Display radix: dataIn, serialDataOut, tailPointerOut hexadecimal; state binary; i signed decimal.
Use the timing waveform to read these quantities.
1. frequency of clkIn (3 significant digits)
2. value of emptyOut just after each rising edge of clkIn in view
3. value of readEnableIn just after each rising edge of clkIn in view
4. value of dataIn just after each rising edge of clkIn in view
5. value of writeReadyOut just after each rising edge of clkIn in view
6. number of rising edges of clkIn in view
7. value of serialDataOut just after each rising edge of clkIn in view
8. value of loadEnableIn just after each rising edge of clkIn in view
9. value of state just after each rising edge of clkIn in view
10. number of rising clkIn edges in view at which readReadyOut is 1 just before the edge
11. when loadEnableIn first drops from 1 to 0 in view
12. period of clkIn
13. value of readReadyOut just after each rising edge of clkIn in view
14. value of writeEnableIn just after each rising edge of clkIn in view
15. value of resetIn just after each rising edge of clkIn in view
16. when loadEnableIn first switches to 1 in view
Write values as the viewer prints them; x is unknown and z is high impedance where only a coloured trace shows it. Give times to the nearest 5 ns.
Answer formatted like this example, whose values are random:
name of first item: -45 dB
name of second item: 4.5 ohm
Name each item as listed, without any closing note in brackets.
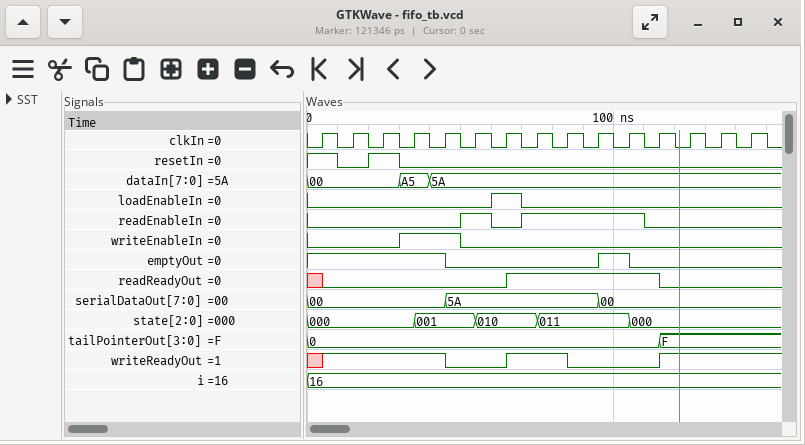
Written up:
frequency of clkIn: 100 MHz
value of emptyOut just after each rising edge of clkIn in view: 1 1 1 1 0 0 0 0 0 1 0 0 0 0 0
value of readEnableIn just after each rising edge of clkIn in view: 0 0 0 0 0 1 0 1 1 1 1 0 0 0 0
value of dataIn just after each rising edge of clkIn in view: 00, 00, 00, A5, 5A, 5A, 5A, 5A, 5A, 5A, 5A, 5A, 5A, 5A, 5A
value of writeReadyOut just after each rising edge of clkIn in view: 1 1 1 1 0 0 1 1 0 0 0 1 1 1 1
number of rising edges of clkIn in view: 15
value of serialDataOut just after each rising edge of clkIn in view: 00, 00, 00, 00, 5A, 5A, 5A, 5A, 5A, 00, 00, 00, 00, 00, 00
value of loadEnableIn just after each rising edge of clkIn in view: 0 0 0 0 0 0 1 0 0 0 0 0 0 0 0
value of state just after each rising edge of clkIn in view: 000, 000, 000, 001, 001, 010, 010, 011, 011, 011, 000, 000, 000, 000, 000
number of rising clkIn edges in view at which readReadyOut is 1 just before the edge: 5
when loadEnableIn first drops from 1 to 0 in view: 70 ns
period of clkIn: 10 ns
value of readReadyOut just after each rising edge of clkIn in view: 0 0 0 0 0 0 1 1 1 1 1 0 0 0 0
value of writeEnableIn just after each rising edge of clkIn in view: 0 0 0 1 1 0 0 0 0 0 0 0 0 0 0
value of resetIn just after each rising edge of clkIn in view: 1 0 1 0 0 0 0 0 0 0 0 0 0 0 0
when loadEnableIn first switches to 1 in view: 60 ns
